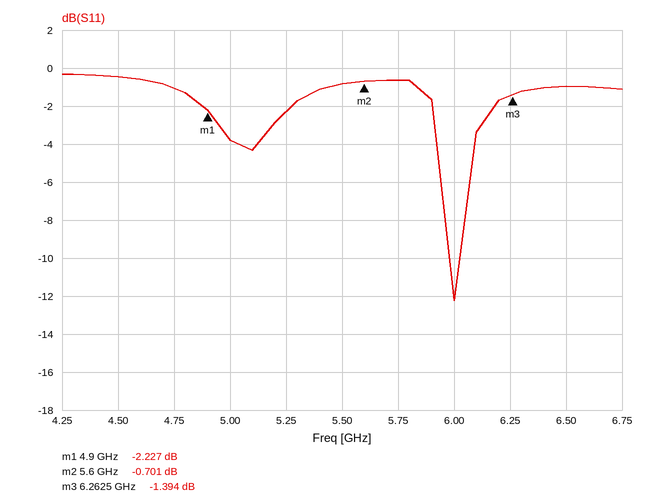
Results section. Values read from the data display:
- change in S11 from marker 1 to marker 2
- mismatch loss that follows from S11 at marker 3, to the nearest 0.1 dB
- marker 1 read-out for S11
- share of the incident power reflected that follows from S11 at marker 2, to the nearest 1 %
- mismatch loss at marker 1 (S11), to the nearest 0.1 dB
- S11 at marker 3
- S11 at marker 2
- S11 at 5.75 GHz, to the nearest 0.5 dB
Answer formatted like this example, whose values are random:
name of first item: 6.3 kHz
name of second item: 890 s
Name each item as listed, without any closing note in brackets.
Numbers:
change in S11 from marker 1 to marker 2: 1.526 dB
mismatch loss that follows from S11 at marker 3, to the nearest 0.1 dB: 5.6 dB
marker 1 read-out for S11: -2.227 dB
share of the incident power reflected that follows from S11 at marker 2, to the nearest 1 %: 85 %
mismatch loss at marker 1 (S11), to the nearest 0.1 dB: 4.0 dB
S11 at marker 3: -1.394 dB
S11 at marker 2: -0.701 dB
S11 at 5.75 GHz, to the nearest 0.5 dB: -0.5 dB
